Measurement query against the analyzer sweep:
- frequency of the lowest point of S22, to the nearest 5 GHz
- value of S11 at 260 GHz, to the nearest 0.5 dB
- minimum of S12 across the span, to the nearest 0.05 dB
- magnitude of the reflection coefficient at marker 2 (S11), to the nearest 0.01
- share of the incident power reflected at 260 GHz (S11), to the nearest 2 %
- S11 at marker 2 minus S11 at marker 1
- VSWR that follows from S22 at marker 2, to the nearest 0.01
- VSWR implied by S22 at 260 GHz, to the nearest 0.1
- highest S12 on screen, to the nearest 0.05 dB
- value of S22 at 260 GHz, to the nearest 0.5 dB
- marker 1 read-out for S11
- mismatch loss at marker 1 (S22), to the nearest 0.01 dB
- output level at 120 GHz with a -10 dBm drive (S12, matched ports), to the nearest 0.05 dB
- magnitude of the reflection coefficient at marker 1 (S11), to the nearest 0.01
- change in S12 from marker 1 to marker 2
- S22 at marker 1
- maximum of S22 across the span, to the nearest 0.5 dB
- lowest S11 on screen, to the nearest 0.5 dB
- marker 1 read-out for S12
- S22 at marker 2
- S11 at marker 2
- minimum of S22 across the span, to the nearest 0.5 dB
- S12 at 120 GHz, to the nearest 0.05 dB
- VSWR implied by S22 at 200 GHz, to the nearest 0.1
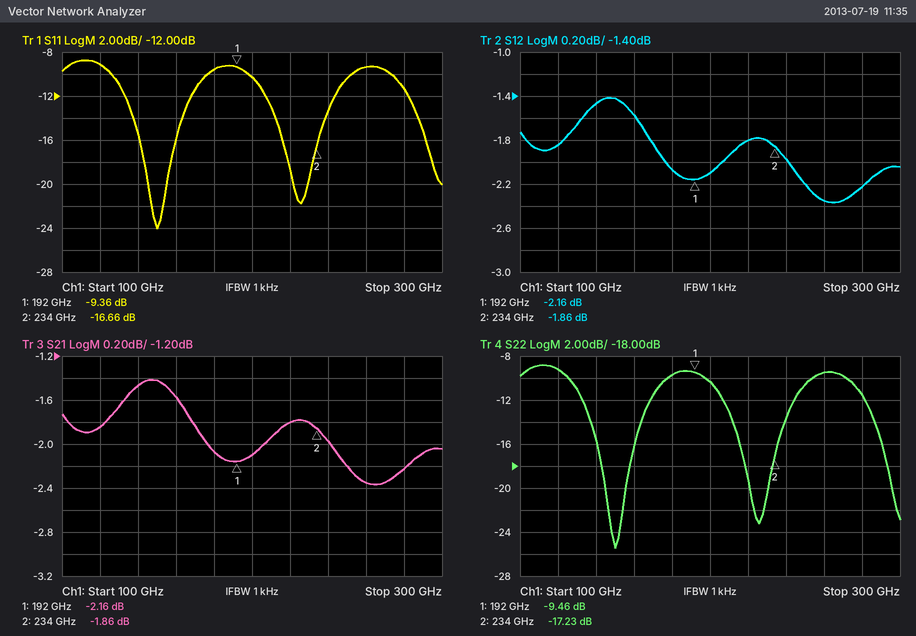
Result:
150 GHz
-9.5 dB
-2.35 dB
0.15
12 %
-7.30 dB
1.32
2.0
-1.40 dB
-9.5 dB
-9.36 dB
0.52 dB
-11.85 dBm
0.34
0.30 dB
-9.46 dB
-9.0 dB
-24.0 dB
-2.16 dB
-17.23 dB
-16.66 dB
-25.5 dB
-1.85 dB
1.9
